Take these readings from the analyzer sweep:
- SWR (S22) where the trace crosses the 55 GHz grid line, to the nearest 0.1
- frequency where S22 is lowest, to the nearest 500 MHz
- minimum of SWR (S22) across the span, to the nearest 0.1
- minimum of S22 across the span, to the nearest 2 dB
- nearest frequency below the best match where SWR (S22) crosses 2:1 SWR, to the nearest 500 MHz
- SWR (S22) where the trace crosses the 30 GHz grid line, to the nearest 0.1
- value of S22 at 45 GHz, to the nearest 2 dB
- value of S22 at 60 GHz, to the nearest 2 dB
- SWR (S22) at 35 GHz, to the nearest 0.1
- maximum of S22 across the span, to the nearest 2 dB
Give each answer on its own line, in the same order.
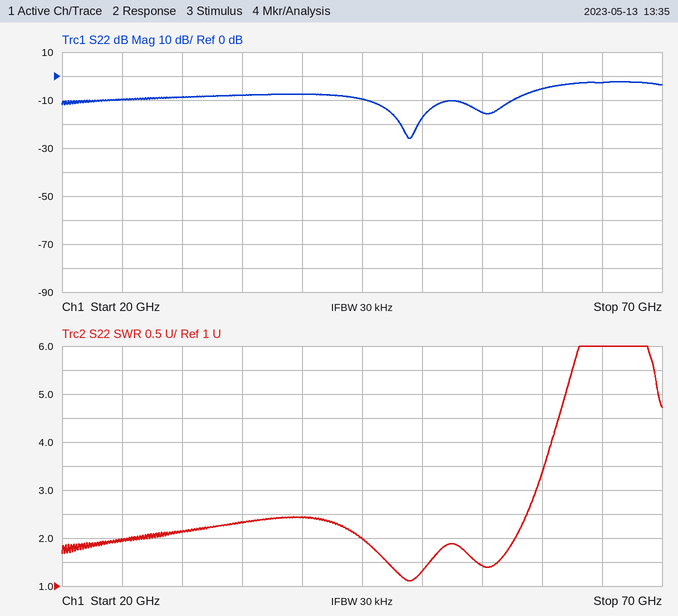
1.4
49.0 GHz
1.1
-26 dB
45.0 GHz
2.1
-10 dB
-6 dB
2.3
-2 dB
